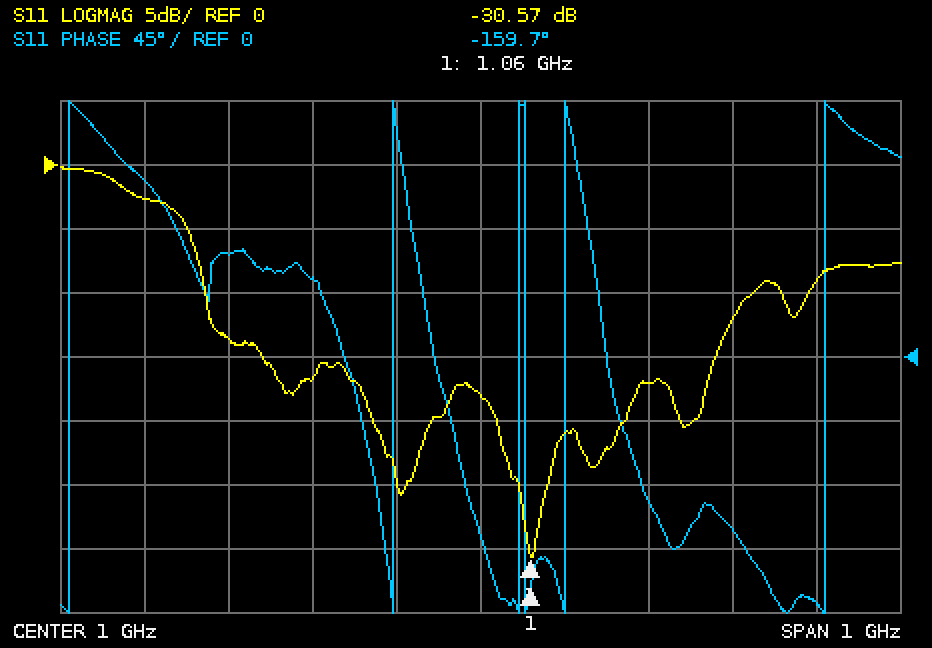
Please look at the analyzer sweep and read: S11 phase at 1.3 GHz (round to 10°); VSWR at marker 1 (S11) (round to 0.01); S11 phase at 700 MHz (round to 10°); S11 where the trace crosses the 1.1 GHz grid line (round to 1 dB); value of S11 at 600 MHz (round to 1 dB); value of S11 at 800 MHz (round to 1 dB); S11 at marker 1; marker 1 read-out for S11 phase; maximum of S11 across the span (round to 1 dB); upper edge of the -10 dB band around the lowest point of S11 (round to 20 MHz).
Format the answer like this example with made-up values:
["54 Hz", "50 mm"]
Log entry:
["-120°", "1.06", "70°", "-21 dB", "-3 dB", "-17 dB", "-30.57 dB", "-159.7°", "0 dB", "1.32 GHz"]
